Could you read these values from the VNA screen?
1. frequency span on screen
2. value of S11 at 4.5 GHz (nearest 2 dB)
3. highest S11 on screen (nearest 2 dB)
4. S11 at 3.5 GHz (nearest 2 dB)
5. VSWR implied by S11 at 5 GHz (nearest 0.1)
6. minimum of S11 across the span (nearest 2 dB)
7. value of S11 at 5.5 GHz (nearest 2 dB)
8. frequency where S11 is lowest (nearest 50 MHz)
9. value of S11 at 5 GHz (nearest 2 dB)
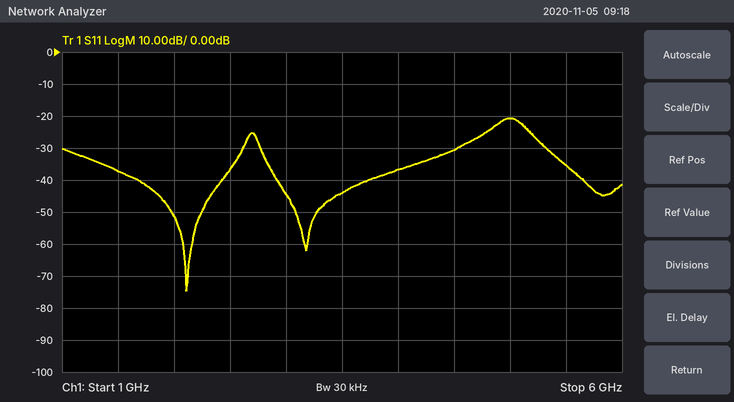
5 GHz
-30 dB
-20 dB
-44 dB
1.2
-74 dB
-36 dB
2.10 GHz
-20 dB
